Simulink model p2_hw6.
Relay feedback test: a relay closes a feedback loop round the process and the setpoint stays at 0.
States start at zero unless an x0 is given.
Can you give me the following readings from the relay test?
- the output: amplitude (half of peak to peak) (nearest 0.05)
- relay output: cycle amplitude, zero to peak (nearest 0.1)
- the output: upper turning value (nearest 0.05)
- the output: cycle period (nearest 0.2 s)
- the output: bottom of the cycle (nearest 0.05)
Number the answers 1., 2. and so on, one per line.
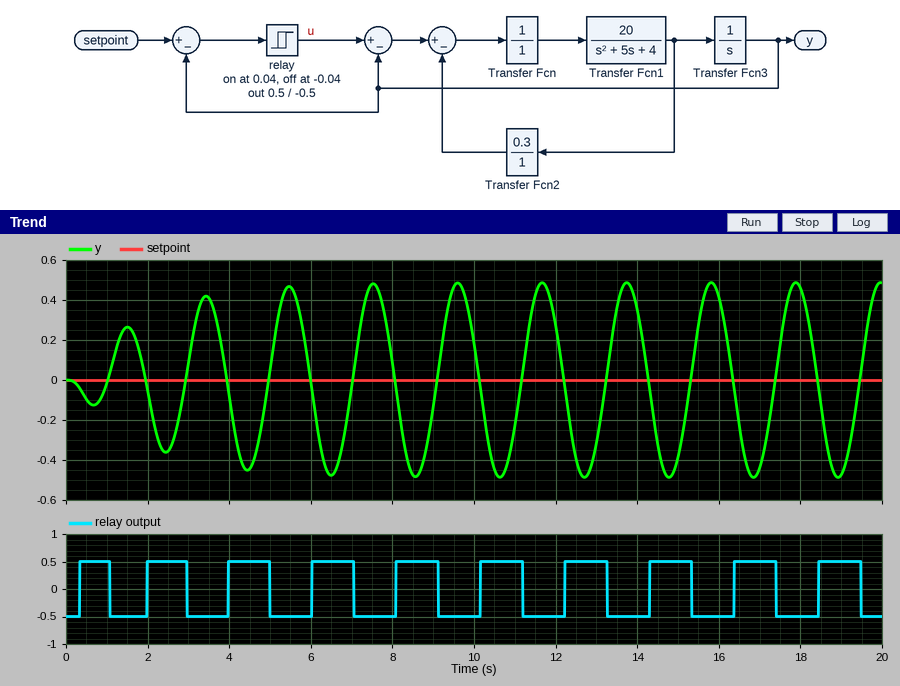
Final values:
1. 0.50
2. 0.5
3. 0.50
4. 2.0 s
5. -0.50
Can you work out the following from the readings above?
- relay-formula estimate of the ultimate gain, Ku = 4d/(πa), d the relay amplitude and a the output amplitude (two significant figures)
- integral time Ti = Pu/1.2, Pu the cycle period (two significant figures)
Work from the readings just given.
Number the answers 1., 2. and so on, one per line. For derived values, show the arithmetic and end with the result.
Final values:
1. 4 × 0.5 / (π × 0.5) = 1.3
2. 2 / 1.2 = 1.7 s
